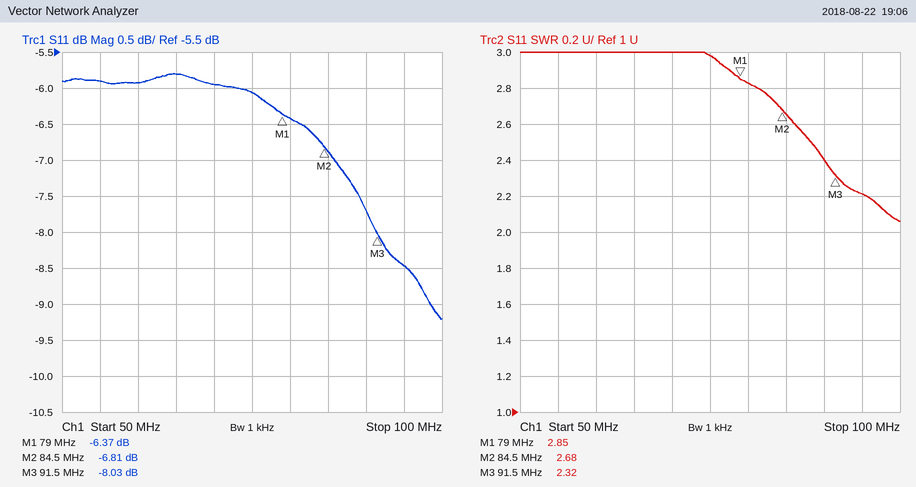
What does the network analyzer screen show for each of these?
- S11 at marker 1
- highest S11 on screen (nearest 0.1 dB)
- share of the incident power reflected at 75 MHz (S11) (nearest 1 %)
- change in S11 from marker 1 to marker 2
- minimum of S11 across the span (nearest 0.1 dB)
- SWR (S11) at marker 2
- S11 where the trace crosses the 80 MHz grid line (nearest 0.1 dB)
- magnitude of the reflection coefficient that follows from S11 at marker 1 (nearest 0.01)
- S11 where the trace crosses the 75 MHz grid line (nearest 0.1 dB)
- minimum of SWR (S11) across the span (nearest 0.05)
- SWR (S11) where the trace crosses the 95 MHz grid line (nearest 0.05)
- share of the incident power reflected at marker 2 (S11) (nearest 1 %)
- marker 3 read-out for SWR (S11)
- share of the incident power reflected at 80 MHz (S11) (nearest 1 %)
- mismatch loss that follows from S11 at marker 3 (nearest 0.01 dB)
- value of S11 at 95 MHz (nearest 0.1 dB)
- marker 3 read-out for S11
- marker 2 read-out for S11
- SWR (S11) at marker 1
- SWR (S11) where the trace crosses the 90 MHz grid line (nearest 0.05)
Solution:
-6.37 dB
-5.8 dB
25 %
-0.44 dB
-9.2 dB
2.68
-6.4 dB
0.48
-6.1 dB
2.05
2.20
21 %
2.32
23 %
0.74 dB
-8.5 dB
-8.03 dB
-6.81 dB
2.85
2.40
